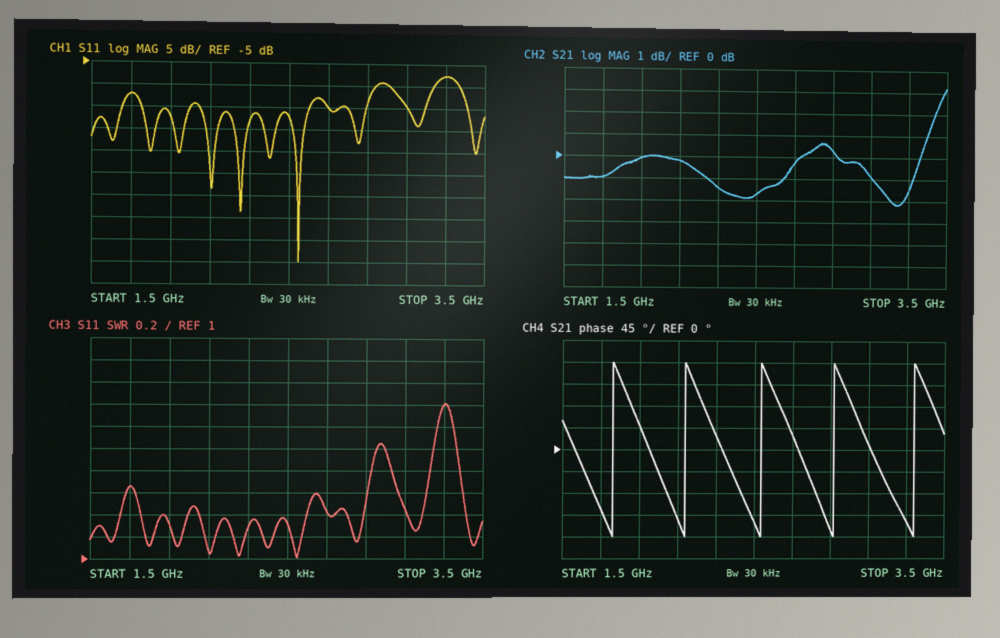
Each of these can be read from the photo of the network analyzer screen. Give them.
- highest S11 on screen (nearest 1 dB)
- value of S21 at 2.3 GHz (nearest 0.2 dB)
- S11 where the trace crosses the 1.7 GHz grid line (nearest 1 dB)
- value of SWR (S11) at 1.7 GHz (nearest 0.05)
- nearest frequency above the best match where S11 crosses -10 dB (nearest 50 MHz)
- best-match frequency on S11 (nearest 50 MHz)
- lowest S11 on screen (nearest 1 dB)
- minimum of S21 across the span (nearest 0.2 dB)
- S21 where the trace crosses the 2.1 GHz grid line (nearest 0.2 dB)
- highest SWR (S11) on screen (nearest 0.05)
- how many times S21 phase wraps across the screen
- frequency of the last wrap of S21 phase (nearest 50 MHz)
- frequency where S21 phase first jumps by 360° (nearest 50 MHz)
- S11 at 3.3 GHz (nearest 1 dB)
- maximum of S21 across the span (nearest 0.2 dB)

-8 dB
-1.4 dB
-12 dB
1.65
2.95 GHz
2.55 GHz
-50 dB
-2.2 dB
-0.2 dB
2.40
5
3.35 GHz
1.75 GHz
-8 dB
3.2 dB
